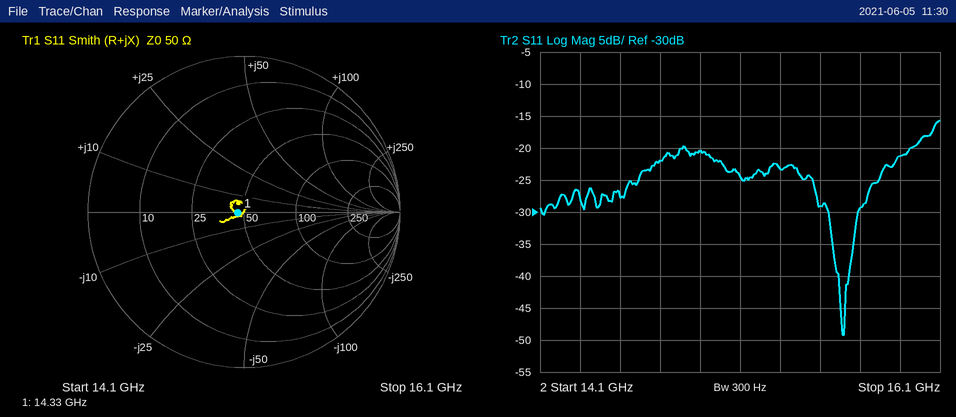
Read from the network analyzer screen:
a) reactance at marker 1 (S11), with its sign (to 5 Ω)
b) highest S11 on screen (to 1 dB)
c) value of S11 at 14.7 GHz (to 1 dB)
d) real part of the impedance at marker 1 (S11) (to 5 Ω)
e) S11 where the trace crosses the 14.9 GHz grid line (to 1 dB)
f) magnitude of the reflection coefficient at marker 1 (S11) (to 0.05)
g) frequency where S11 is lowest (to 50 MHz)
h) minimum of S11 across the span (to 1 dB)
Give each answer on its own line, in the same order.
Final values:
0 Ω
-16 dB
-22 dB
45 Ω
-20 dB
0.05
15.60 GHz
-49 dB
